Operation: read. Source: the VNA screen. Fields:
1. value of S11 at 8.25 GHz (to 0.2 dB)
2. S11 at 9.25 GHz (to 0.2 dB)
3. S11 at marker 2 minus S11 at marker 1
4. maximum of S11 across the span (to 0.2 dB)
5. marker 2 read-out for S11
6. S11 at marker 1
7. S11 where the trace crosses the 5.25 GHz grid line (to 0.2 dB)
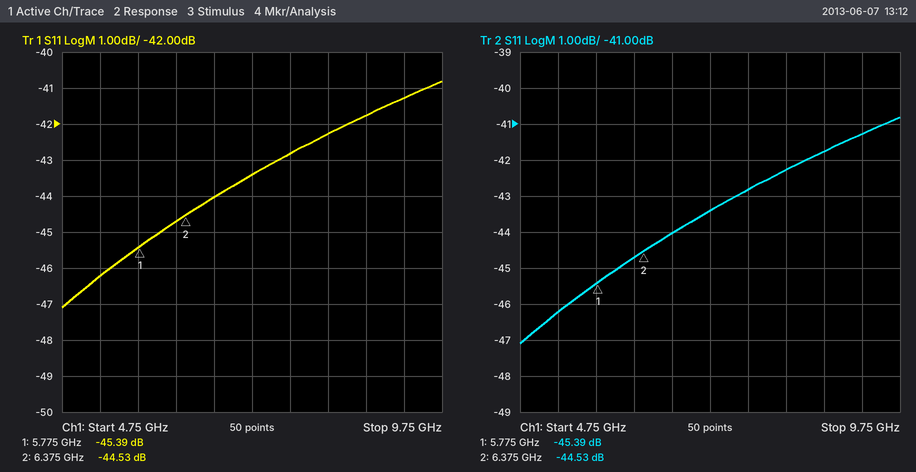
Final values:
-42.2 dB
-41.2 dB
0.86 dB
-40.8 dB
-44.53 dB
-45.39 dB
-46.2 dB
